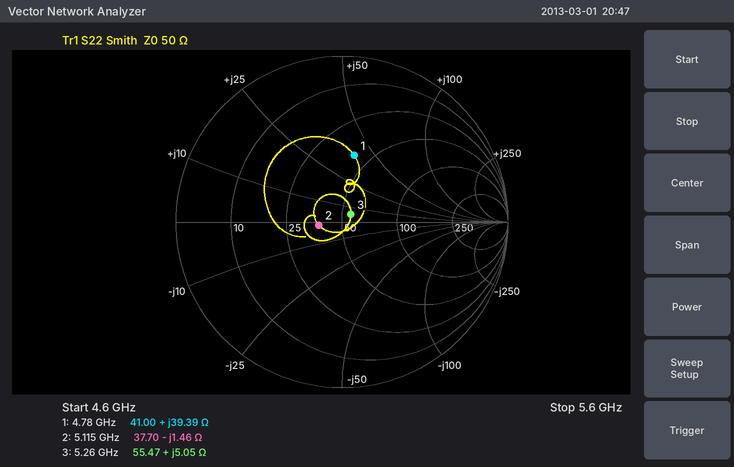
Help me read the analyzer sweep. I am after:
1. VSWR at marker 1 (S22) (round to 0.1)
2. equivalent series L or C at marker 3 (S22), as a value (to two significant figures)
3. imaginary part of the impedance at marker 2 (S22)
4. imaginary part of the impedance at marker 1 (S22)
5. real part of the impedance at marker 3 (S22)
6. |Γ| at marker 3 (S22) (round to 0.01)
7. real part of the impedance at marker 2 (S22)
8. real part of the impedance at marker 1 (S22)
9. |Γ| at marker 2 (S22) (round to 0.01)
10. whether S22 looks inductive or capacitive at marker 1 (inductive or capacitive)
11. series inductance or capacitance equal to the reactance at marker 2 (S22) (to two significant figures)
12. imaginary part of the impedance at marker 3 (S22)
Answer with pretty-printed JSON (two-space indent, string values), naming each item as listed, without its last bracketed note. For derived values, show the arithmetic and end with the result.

{
  "VSWR at marker 1 (S22)": "2.4",
  "equivalent series L or C at marker 3 (S22), as a value": "L = 5.05 Ω/(2π × 5.26 GHz) ≈ 153 pH, so 150 pH to two significant figures",
  "imaginary part of the impedance at marker 2": "-1.46 Ω",
  "imaginary part of the impedance at marker 1": "+39.39 Ω",
  "real part of the impedance at marker 3": "55.47 Ω",
  "|Γ| at marker 3 (S22)": "0.07",
  "real part of the impedance at marker 2": "37.70 Ω",
  "real part of the impedance at marker 1": "41.00 Ω",
  "|Γ| at marker 2 (S22)": "0.14",
  "whether S22 looks inductive or capacitive at marker 1": "inductive",
  "series inductance or capacitance equal to the reactance at marker 2 (S22)": "C = 1/(2π × 5.115 GHz × 1.46 Ω) ≈ 21 pF",
  "imaginary part of the impedance at marker 3": "+5.05 Ω"
}
